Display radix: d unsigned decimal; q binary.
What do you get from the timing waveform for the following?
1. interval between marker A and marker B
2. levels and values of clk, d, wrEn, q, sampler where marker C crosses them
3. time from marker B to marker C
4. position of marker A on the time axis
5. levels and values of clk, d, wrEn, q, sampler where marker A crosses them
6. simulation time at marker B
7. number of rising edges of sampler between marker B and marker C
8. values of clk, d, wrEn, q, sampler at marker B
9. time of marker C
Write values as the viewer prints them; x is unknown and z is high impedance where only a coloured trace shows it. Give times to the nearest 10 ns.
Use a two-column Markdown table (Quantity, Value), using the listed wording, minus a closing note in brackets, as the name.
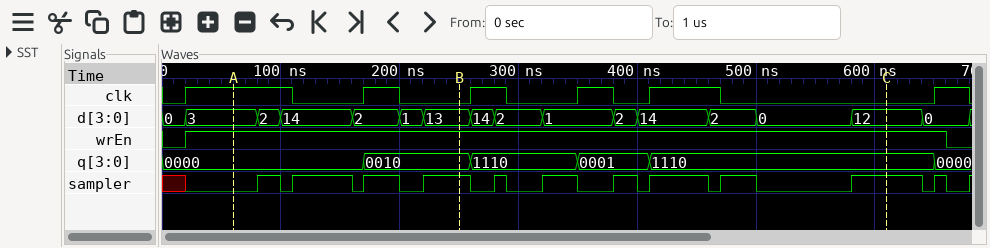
| Quantity | Value |
|---|---|
| interval between marker A and marker B | 190 ns |
| levels and values of clk, d, wrEn, q, sampler where marker C crosses them | clk=0, d=12, wrEn=1, q=1110, sampler=1 |
| time from marker B to marker C | 360 ns |
| position of marker A on the time axis | 60 ns |
| levels and values of clk, d, wrEn, q, sampler where marker A crosses them | clk=1, d=3, wrEn=1, q=0000, sampler=0 |
| simulation time at marker B | 250 ns |
| number of rising edges of sampler between marker B and marker C | 6 |
| values of clk, d, wrEn, q, sampler at marker B | clk=0, d=13, wrEn=1, q=0010, sampler=1 |
| time of marker C | 610 ns |
